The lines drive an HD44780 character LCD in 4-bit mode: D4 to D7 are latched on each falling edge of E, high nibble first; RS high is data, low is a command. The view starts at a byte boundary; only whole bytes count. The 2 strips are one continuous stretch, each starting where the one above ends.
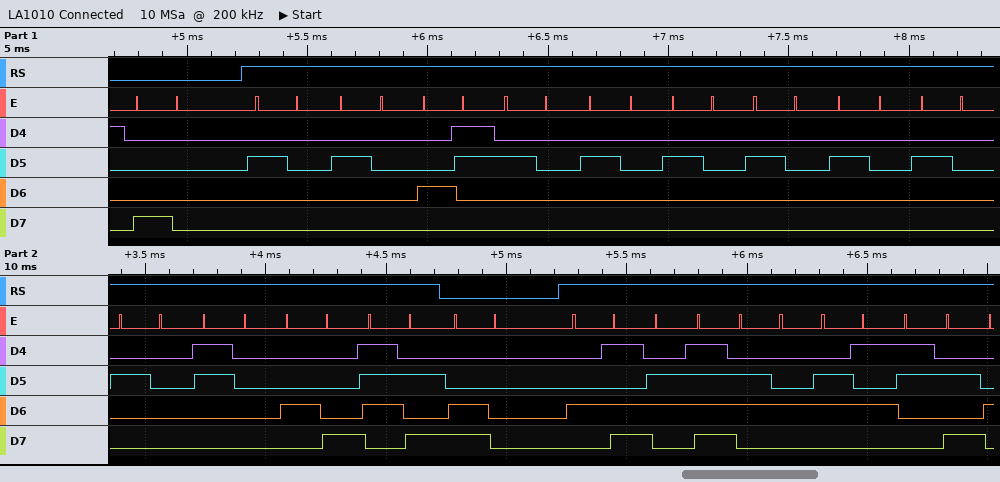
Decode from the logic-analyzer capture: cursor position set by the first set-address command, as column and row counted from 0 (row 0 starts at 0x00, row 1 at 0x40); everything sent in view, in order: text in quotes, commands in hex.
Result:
column 0, row 0
0x80 "  C       0Hz" 0xC0 "Mode:"
